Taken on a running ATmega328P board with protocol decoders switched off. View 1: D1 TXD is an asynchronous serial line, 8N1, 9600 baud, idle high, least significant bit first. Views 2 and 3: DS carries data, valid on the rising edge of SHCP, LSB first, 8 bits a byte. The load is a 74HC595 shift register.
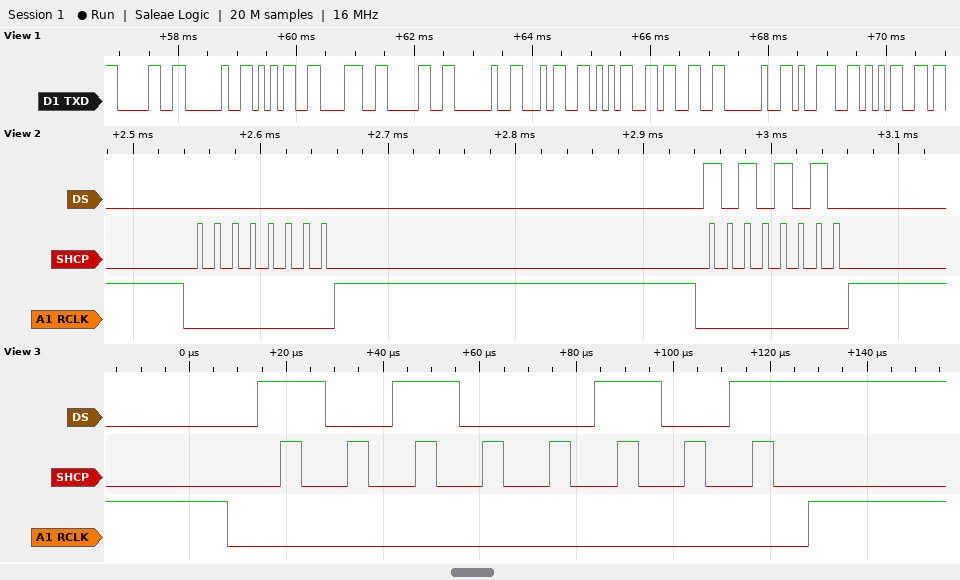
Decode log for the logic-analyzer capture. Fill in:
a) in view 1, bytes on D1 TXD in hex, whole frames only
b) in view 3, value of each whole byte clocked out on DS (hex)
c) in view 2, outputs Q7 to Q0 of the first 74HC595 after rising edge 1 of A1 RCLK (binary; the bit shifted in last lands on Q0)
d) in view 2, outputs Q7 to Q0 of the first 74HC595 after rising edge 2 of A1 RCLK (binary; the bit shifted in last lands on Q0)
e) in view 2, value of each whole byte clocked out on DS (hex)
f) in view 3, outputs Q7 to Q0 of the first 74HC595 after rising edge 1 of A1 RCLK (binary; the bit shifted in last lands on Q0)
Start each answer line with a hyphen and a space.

- 30 20 35 38 30 20 34 35 33 20 39 35
- A5
- 00000000
- 10101010
- 00 55
- 10100101
